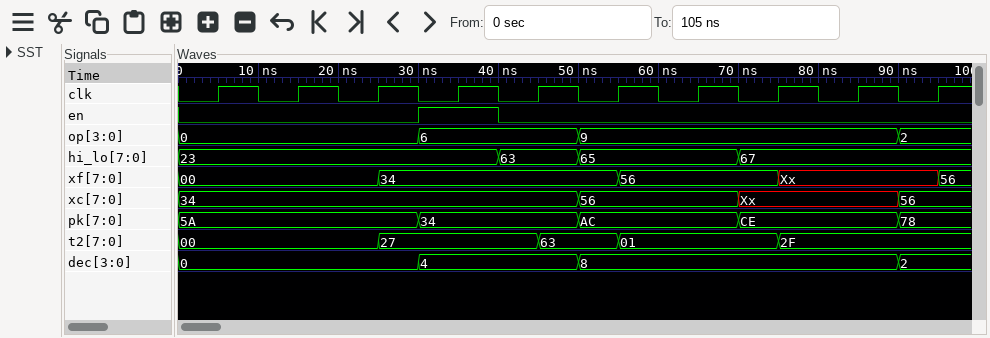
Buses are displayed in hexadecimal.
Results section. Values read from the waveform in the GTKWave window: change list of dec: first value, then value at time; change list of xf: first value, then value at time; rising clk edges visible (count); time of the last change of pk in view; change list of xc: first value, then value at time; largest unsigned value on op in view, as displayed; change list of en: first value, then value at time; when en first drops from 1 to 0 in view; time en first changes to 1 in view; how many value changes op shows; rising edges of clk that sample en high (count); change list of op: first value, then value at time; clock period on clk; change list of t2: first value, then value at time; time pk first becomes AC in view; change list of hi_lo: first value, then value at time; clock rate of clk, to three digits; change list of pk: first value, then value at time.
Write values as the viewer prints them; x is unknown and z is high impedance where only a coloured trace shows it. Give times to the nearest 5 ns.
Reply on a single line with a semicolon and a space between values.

0, 4 at 30 ns, 8 at 50 ns, 2 at 90 ns; 00, 34 at 25 ns, 56 at 55 ns, Xx at 75 ns, 56 at 95 ns; 10; 90 ns; 34, 56 at 50 ns, Xx at 70 ns, 56 at 90 ns; 9; 0, 1 at 30 ns, 0 at 40 ns; 40 ns; 30 ns; 3; 1; 0, 6 at 30 ns, 9 at 50 ns, 2 at 90 ns; 10 ns; 00, 27 at 25 ns, 63 at 45 ns, 01 at 55 ns, 2F at 75 ns; 50 ns; 23, 63 at 40 ns, 65 at 50 ns, 67 at 70 ns; 100 MHz; 5A, 34 at 30 ns, AC at 50 ns, CE at 70 ns, 78 at 90 ns
